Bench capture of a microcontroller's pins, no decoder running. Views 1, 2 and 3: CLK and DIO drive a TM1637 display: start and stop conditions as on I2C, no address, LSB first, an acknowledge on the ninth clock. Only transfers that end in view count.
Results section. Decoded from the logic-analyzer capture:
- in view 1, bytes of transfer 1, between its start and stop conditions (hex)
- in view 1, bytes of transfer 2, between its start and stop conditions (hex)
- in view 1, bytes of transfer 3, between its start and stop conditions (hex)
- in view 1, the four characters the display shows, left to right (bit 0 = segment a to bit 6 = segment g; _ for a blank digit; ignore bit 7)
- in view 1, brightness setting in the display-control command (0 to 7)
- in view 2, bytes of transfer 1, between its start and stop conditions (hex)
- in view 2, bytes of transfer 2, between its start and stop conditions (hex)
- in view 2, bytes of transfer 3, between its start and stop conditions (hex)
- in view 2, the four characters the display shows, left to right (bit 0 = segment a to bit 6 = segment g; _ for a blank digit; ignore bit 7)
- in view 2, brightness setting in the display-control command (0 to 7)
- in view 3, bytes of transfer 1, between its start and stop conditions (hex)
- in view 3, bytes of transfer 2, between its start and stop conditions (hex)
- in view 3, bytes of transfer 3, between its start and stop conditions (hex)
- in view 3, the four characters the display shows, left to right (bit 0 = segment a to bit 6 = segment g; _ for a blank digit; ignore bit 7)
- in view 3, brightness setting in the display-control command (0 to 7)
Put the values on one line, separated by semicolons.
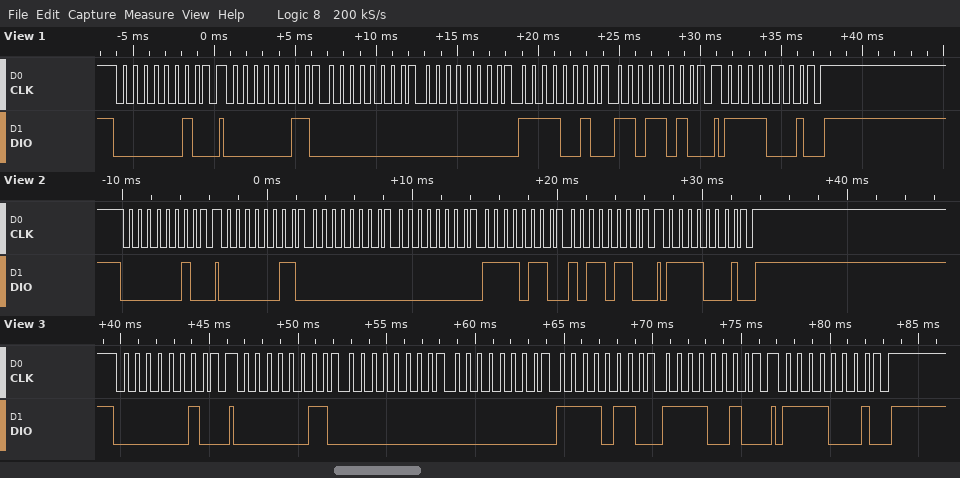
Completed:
40; C0 00 00 4F 5B; 8F; __32; 7; 40; C0 00 00 6F 6D; 8F; __95; 7; 40; C0 00 00 6F 4F; 8F; __93; 7
